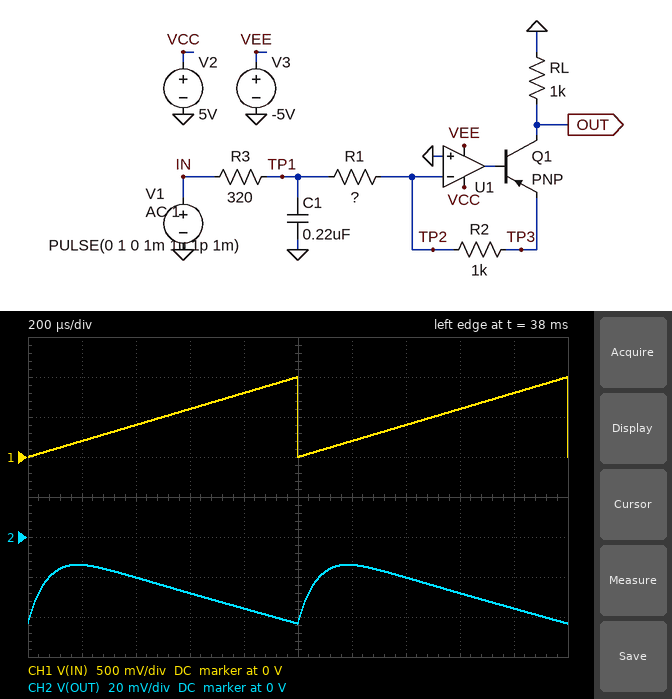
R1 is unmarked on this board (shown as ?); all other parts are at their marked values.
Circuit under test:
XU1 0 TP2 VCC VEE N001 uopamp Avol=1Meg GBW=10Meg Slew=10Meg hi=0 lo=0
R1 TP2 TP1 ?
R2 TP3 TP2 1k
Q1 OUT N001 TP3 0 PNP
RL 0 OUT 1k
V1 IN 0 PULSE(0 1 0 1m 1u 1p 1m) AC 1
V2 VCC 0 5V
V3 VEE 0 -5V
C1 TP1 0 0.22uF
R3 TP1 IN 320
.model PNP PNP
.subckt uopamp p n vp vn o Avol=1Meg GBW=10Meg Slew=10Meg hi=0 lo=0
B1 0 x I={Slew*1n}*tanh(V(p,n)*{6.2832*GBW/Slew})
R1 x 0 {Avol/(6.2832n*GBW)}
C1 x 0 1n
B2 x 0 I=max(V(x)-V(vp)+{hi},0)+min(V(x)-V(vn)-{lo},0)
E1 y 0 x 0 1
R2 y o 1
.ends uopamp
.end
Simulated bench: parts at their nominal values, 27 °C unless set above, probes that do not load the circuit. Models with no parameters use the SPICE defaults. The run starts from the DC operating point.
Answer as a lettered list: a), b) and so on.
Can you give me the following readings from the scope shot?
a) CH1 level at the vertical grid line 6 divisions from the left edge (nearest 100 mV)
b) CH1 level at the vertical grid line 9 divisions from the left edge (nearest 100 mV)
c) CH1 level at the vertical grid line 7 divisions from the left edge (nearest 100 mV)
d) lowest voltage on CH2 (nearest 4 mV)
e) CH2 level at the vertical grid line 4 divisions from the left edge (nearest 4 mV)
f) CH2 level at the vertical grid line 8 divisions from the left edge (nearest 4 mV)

a) 200 mV
b) 800 mV
c) 400 mV
d) -44 mV
e) -36 mV
f) -28 mV
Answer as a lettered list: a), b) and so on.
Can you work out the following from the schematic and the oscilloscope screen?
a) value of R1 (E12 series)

a) 27 kΩ
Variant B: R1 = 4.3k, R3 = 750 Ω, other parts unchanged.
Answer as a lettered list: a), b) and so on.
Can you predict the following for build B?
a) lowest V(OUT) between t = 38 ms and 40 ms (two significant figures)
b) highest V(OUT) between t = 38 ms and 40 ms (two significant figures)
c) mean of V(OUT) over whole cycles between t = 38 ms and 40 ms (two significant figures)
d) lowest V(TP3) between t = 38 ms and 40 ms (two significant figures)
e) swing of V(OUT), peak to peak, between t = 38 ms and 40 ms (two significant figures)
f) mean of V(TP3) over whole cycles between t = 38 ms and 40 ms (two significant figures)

a) -180 mV
b) -64 mV
c) -110 mV
d) -170 mV
e) 120 mV
f) -99 mV
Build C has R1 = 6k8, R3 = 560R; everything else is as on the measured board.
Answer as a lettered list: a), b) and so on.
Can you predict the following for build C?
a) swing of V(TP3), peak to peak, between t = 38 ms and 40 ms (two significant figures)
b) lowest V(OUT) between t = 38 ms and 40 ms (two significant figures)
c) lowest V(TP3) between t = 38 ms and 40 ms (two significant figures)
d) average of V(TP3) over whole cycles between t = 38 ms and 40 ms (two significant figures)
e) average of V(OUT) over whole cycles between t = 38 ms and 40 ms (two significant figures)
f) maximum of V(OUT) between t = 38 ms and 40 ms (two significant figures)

a) 87 mV
b) -130 mV
c) -120 mV
d) -68 mV
e) -78 mV
f) -43 mV
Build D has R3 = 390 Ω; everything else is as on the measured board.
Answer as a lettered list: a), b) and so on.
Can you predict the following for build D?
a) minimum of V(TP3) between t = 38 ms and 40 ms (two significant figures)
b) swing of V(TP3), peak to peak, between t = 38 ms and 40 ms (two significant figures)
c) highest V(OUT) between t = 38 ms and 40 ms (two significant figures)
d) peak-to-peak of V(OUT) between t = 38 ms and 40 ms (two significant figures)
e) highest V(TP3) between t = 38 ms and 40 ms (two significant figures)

a) -33 mV
b) 26 mV
c) -15 mV
d) 28 mV
e) -7.6 mV
